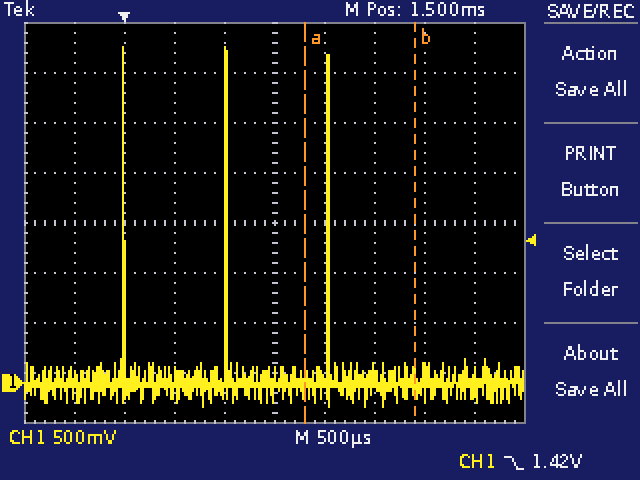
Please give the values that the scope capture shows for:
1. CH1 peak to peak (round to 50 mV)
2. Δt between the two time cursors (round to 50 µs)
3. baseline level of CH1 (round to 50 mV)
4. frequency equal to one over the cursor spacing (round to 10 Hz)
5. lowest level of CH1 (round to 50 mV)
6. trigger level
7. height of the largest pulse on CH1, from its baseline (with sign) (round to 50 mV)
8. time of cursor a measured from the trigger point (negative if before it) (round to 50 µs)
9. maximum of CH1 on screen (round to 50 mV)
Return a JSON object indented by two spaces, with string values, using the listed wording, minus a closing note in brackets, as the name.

{
  "CH1 peak to peak": "3.60 V",
  "Δt between the two time cursors": "1.10 ms",
  "baseline level of CH1": "0 mV",
  "frequency equal to one over the cursor spacing": "910 Hz",
  "lowest level of CH1": "-250 mV",
  "trigger level": "1.42 V",
  "height of the largest pulse on CH1, from its baseline (with sign)": "+3.35 V",
  "time of cursor a measured from the trigger point (negative if before it)": "+1.80 ms",
  "maximum of CH1 on screen": "3.35 V"
}
